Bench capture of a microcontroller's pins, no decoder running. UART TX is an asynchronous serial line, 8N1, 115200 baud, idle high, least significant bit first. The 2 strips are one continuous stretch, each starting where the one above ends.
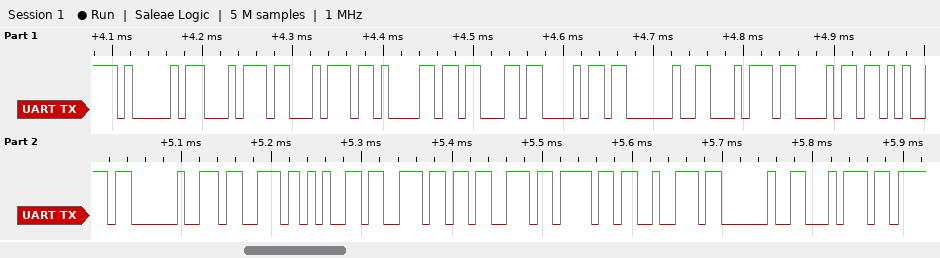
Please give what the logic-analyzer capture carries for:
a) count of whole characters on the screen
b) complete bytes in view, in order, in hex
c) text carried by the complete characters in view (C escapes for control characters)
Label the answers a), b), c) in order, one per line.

a) 19
b) 41 74 74 61 63 68 20 74 68 65 20 73 65 6E 73 6F 72 20 74
c) "Attach the sensor t"
